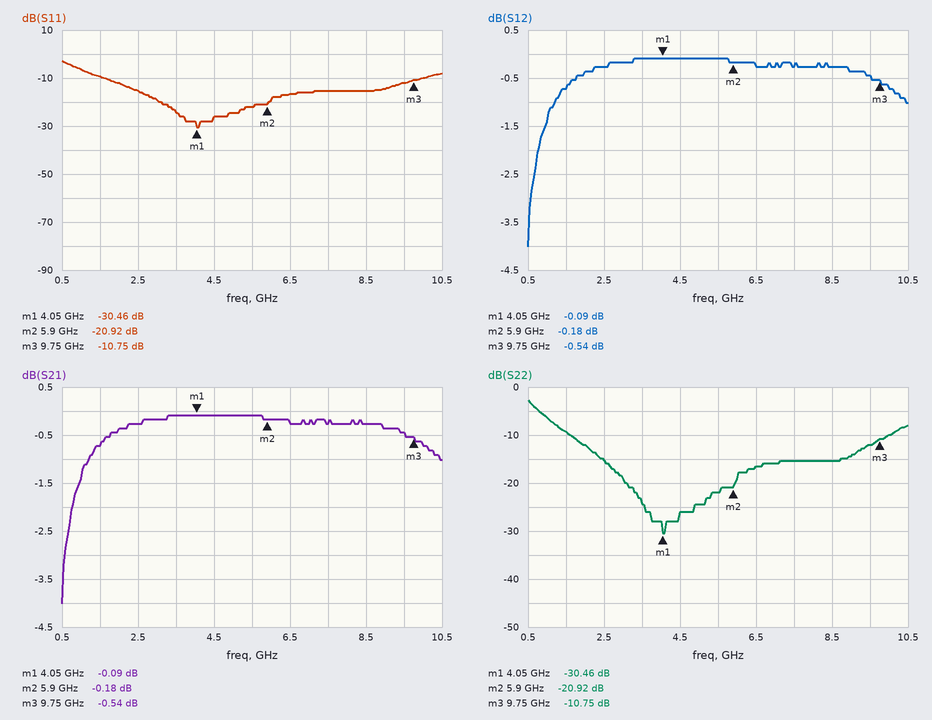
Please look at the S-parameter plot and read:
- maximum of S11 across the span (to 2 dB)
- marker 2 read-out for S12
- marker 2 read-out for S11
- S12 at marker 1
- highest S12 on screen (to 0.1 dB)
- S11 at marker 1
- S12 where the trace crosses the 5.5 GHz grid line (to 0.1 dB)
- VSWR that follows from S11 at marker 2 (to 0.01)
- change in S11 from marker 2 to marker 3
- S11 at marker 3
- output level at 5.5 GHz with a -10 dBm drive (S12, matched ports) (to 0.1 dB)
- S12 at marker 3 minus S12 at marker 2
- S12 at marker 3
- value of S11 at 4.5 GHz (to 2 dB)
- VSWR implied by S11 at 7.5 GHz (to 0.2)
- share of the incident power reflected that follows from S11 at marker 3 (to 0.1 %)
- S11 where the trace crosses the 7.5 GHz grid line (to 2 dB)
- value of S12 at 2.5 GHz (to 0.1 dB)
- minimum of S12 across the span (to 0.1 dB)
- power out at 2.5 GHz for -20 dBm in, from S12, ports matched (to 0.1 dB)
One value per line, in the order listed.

-2 dB
-0.18 dB
-20.92 dB
-0.09 dB
-0.1 dB
-30.46 dB
-0.1 dB
1.20
10.17 dB
-10.75 dB
-10.1 dBm
-0.36 dB
-0.54 dB
-26 dB
1.4
8.4 %
-16 dB
-0.3 dB
-4.0 dB
-20.3 dBm
